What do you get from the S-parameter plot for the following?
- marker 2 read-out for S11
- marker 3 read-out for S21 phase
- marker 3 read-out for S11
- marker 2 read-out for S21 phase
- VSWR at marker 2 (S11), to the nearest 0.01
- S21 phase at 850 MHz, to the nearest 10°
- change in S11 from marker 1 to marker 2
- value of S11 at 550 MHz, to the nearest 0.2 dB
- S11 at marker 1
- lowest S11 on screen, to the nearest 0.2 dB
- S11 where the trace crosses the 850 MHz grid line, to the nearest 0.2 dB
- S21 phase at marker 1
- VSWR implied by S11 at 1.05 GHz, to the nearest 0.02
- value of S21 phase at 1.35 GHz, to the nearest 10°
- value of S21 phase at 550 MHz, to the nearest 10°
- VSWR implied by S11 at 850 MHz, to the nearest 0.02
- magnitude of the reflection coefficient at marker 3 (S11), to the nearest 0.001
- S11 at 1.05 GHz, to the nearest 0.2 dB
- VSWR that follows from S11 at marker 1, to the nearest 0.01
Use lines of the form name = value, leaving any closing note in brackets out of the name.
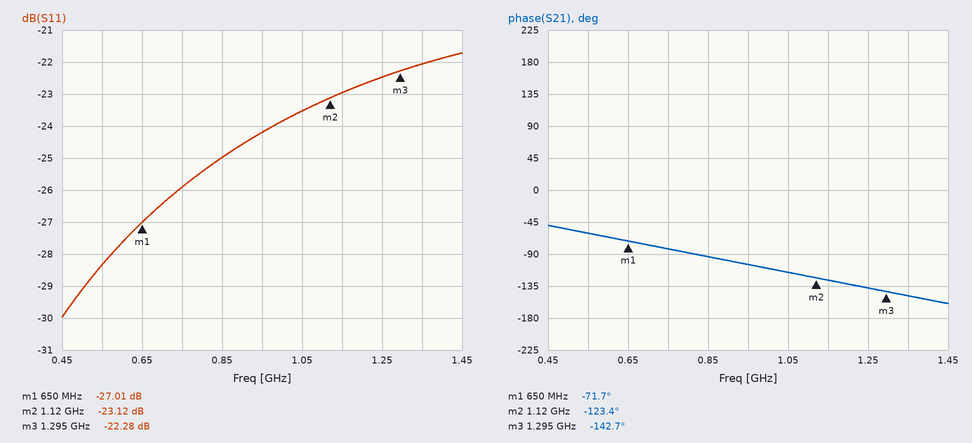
marker 2 read-out for S11 = -23.12 dB
marker 3 read-out for S21 phase = -142.7°
marker 3 read-out for S11 = -22.28 dB
marker 2 read-out for S21 phase = -123.4°
VSWR at marker 2 (S11), to the nearest 0.01 = 1.15
S21 phase at 850 MHz, to the nearest 10° = -90°
change in S11 from marker 1 to marker 2 = 3.89 dB
value of S11 at 550 MHz, to the nearest 0.2 dB = -28.4 dB
S11 at marker 1 = -27.01 dB
lowest S11 on screen, to the nearest 0.2 dB = -30.0 dB
S11 where the trace crosses the 850 MHz grid line, to the nearest 0.2 dB = -25.0 dB
S21 phase at marker 1 = -71.7°
VSWR implied by S11 at 1.05 GHz, to the nearest 0.02 = 1.14
value of S21 phase at 1.35 GHz, to the nearest 10° = -150°
value of S21 phase at 550 MHz, to the nearest 10° = -60°
VSWR implied by S11 at 850 MHz, to the nearest 0.02 = 1.12
magnitude of the reflection coefficient at marker 3 (S11), to the nearest 0.001 = 0.077
S11 at 1.05 GHz, to the nearest 0.2 dB = -23.6 dB
VSWR that follows from S11 at marker 1, to the nearest 0.01 = 1.09
